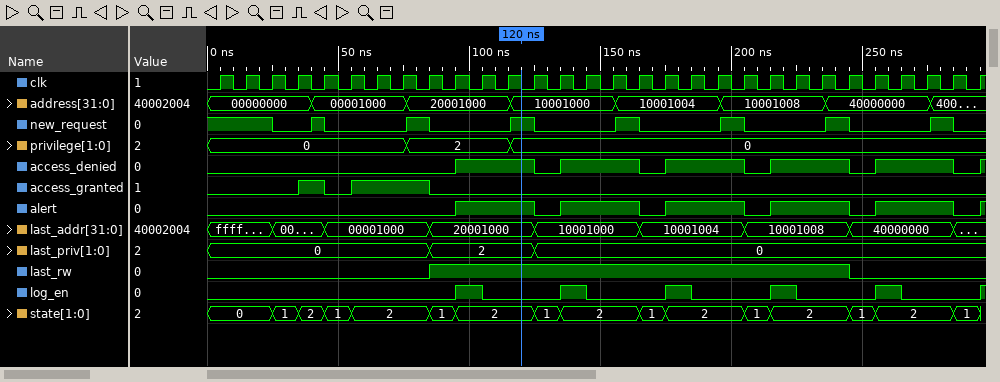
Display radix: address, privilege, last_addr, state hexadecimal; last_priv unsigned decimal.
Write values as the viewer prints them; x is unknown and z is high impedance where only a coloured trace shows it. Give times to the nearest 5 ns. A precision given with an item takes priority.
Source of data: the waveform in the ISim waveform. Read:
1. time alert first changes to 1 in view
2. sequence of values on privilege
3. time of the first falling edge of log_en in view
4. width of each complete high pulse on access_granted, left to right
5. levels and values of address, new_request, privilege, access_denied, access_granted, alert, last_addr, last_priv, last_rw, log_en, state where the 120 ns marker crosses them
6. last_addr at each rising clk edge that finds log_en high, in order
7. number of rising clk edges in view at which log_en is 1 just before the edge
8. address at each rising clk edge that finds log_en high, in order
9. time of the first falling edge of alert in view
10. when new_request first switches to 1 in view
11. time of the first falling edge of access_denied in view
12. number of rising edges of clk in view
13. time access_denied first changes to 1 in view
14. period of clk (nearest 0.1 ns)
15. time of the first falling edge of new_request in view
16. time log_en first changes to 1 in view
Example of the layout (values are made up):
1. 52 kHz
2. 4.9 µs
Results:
1. 95 ns
2. 0, 2, 0
3. 105 ns
4. 10 ns, 30 ns
5. address=10001000, new_request=1, privilege=0, access_denied=1, access_granted=0, alert=1, last_addr=20001000, last_priv=2, last_rw=1, log_en=0, state=2
6. 20001000, 10001000, 10001004, 10001008, 40000000
7. 5
8. 20001000, 10001000, 10001004, 10001008, 40000000
9. 125 ns
10. 40 ns
11. 125 ns
12. 30
13. 95 ns
14. 10 ns
15. 25 ns
16. 95 ns
